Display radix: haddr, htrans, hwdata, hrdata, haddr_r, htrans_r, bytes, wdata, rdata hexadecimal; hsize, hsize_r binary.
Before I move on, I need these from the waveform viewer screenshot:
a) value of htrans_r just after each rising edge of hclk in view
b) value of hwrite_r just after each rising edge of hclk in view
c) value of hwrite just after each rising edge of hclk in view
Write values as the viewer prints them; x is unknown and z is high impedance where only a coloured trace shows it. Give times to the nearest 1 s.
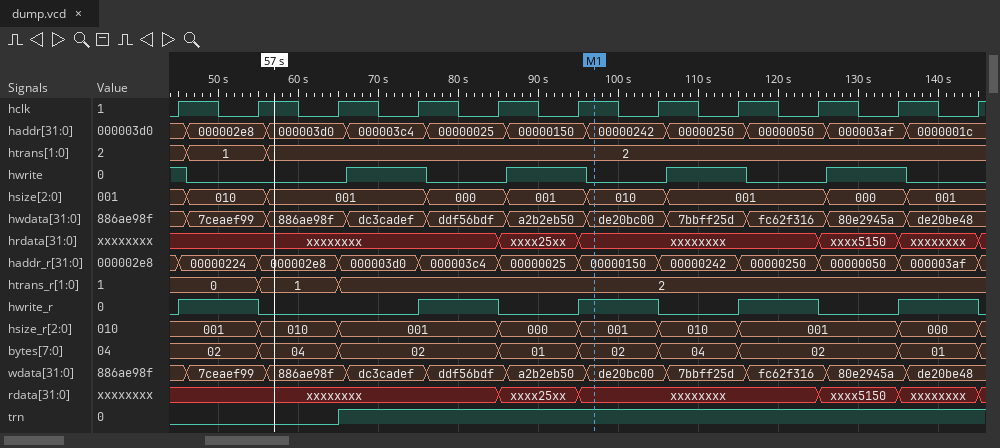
0, 1, 2, 2, 2, 2, 2, 2, 2, 2, 2
1 0 0 1 0 1 0 1 0 1 0
1 0 0 1 0 1 0 1 0 1 0
